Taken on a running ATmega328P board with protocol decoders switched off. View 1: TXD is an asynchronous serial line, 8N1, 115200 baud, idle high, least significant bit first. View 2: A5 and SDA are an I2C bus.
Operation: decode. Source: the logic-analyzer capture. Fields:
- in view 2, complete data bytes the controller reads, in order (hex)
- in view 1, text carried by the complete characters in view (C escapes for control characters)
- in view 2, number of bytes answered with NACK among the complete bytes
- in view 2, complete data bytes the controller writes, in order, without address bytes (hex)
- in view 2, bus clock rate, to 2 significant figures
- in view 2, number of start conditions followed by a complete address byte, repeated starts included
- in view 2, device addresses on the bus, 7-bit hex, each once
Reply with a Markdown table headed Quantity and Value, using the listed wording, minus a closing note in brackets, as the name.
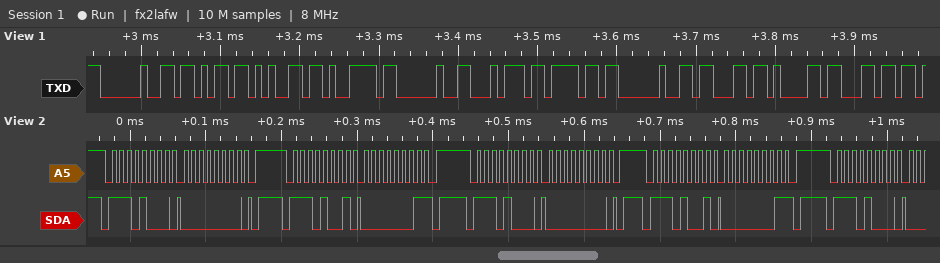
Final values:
| Quantity | Value |
|---|---|
| in view 2, complete data bytes the controller reads, in order | 01 01 |
| in view 1, text carried by the complete characters in view | " key to cal" |
| in view 2, number of bytes answered with NACK among the complete bytes | 2 |
| in view 2, complete data bytes the controller writes, in order, without address bytes | 00 00 |
| in view 2, bus clock rate, to 2 significant figures | 100 kHz |
| in view 2, number of start conditions followed by a complete address byte, repeated starts included | 5 |
| in view 2, device addresses on the bus, 7-bit hex, each once | 0x74 |
